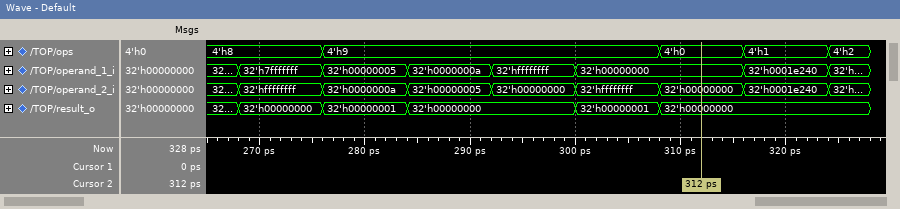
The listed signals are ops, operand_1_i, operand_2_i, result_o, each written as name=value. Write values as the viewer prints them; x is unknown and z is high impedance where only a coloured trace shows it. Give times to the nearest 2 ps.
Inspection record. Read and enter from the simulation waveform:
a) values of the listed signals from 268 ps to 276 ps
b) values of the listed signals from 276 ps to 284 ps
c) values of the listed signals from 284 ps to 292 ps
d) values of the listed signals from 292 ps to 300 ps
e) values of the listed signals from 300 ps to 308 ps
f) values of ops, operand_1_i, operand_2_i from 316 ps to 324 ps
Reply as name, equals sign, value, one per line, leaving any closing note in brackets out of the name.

values of the listed signals from 268 ps to 276 ps = ops=4'h8, operand_1_i=32'h7fffffff, operand_2_i=32'hffffffff, result_o=32'h00000000
values of the listed signals from 276 ps to 284 ps = ops=4'h9, operand_1_i=32'h00000005, operand_2_i=32'h0000000a, result_o=32'h00000001
values of the listed signals from 284 ps to 292 ps = ops=4'h9, operand_1_i=32'h0000000a, operand_2_i=32'h00000005, result_o=32'h00000000
values of the listed signals from 292 ps to 300 ps = ops=4'h9, operand_1_i=32'hffffffff, operand_2_i=32'h00000000, result_o=32'h00000000
values of the listed signals from 300 ps to 308 ps = ops=4'h9, operand_1_i=32'h00000000, operand_2_i=32'hffffffff, result_o=32'h00000001
values of ops, operand_1_i, operand_2_i from 316 ps to 324 ps = ops=4'h1, operand_1_i=32'h0001e240, operand_2_i=32'h0001e240
